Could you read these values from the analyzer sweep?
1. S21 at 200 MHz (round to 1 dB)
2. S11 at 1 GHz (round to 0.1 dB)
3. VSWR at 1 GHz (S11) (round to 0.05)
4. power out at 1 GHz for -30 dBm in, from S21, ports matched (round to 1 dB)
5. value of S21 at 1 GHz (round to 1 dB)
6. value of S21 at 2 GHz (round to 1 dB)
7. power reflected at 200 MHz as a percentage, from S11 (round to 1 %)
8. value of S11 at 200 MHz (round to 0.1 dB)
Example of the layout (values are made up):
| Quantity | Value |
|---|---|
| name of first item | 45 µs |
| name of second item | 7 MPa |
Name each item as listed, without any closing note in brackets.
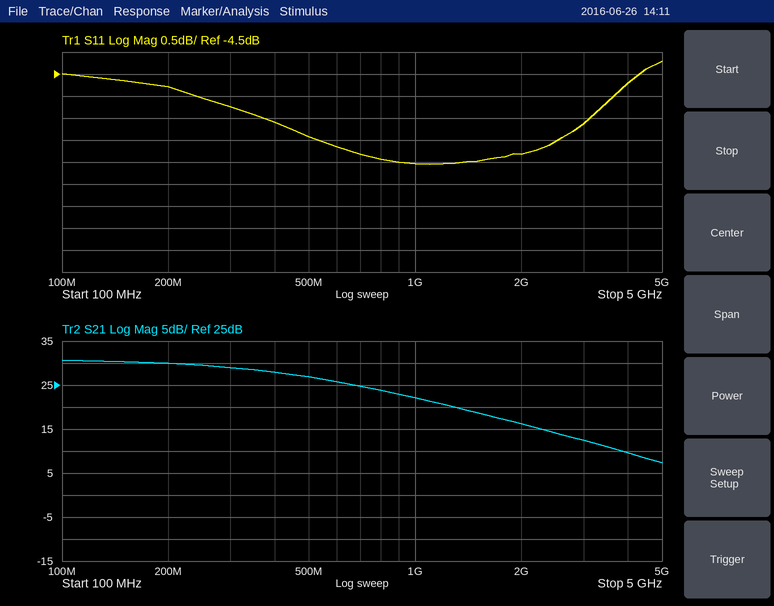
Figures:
| Quantity | Value |
|---|---|
| S21 at 200 MHz | 30 dB |
| S11 at 1 GHz | -6.5 dB |
| VSWR at 1 GHz (S11) | 2.80 |
| power out at 1 GHz for -30 dBm in, from S21, ports matched | -8 dBm |
| value of S21 at 1 GHz | 22 dB |
| value of S21 at 2 GHz | 16 dB |
| power reflected at 200 MHz as a percentage, from S11 | 33 % |
| value of S11 at 200 MHz | -4.8 dB |
